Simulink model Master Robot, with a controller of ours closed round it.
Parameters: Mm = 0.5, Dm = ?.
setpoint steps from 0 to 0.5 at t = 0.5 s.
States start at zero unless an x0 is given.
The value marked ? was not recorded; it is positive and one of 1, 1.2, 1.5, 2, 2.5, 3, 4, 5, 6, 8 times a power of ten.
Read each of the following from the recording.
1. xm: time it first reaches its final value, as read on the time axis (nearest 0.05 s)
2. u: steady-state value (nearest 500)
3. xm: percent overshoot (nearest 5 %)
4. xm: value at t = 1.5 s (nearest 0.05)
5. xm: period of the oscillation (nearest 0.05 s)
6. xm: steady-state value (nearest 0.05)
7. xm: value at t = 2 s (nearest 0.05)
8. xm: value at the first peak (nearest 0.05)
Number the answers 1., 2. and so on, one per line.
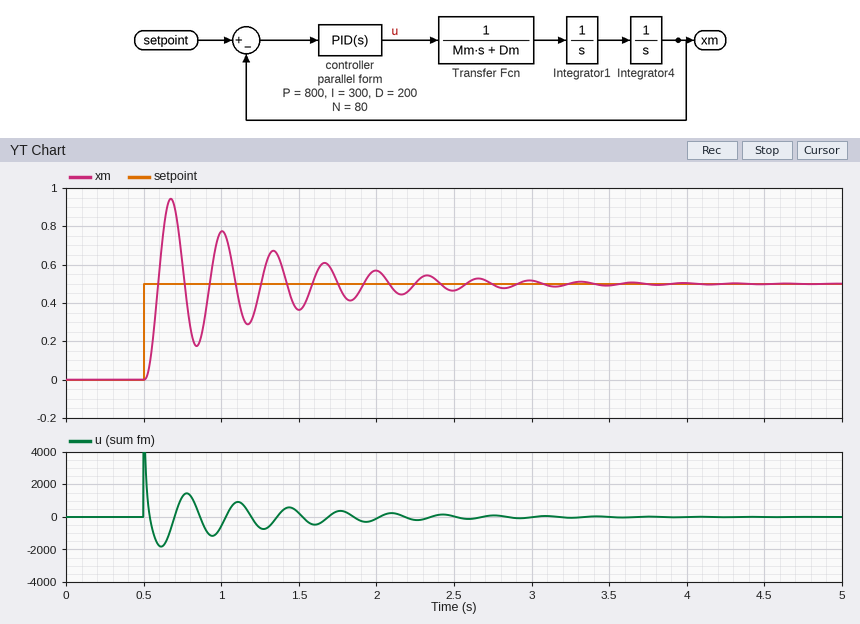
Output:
1. 0.60 s
2. 0
3. 90 %
4. 0.35
5. 0.35 s
6. 0.50
7. 0.55
8. 0.95
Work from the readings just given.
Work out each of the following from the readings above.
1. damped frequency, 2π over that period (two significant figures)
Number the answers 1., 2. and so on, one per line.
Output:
1. 18 rad/s
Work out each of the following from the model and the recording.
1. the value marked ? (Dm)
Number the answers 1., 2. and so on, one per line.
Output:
1. 6
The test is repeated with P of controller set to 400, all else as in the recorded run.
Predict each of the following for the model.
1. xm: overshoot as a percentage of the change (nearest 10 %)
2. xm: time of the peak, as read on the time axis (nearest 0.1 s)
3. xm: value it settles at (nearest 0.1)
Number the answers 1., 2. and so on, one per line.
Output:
1. 70 %
2. 0.7 s
3. 0.5
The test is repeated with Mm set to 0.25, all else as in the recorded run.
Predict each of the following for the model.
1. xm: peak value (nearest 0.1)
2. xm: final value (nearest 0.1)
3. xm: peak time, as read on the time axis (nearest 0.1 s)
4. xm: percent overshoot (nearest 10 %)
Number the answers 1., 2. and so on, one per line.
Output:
1. 0.8
2. 0.5
3. 0.6 s
4. 70 %
